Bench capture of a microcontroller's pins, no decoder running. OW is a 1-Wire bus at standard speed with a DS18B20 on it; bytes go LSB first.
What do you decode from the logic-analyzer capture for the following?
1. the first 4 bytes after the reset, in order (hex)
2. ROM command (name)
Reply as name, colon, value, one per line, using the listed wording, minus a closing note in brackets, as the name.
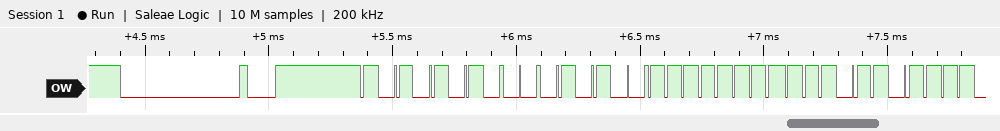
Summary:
the first 4 bytes after the reset, in order: 55 28 FF B7
ROM command: Match ROM
